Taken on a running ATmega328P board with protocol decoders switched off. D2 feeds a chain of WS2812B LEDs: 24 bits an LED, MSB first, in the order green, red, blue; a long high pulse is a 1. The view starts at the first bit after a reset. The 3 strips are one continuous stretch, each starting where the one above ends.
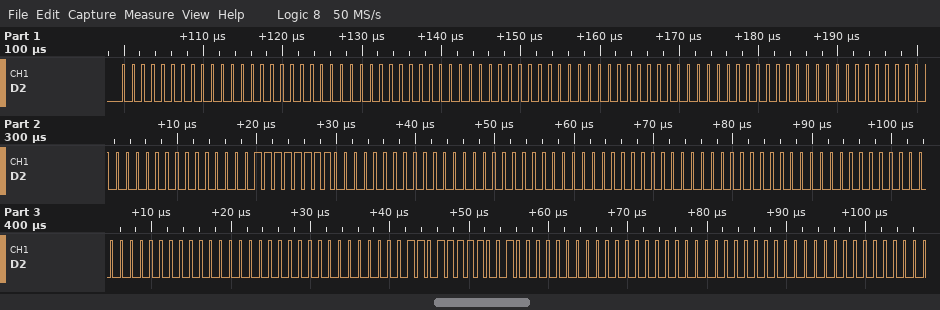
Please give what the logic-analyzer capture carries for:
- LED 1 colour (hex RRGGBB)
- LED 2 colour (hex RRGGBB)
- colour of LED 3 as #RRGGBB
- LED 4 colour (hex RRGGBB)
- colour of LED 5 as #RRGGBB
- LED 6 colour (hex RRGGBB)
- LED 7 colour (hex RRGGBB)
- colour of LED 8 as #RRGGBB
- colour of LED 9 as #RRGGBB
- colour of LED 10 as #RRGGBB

#000000
#000000
#000000
#000000
#00FF00
#000000
#000000
#000000
#C83700
#000000
